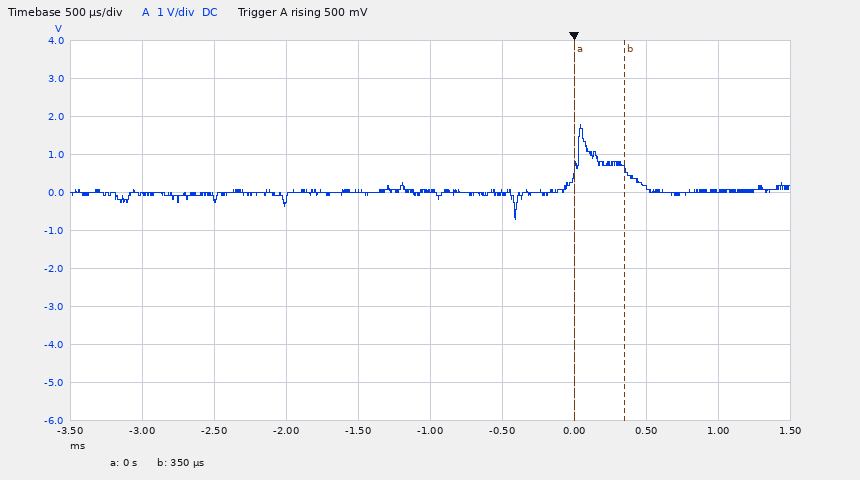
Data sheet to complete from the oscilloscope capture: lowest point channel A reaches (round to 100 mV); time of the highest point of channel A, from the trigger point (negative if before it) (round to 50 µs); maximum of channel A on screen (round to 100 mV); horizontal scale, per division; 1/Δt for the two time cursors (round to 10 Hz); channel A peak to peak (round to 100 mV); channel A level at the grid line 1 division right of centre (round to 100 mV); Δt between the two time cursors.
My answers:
-700 mV
+50 µs
1.8 V
500 µs
2.86 kHz
2.5 V
0.0 V
350 µs
